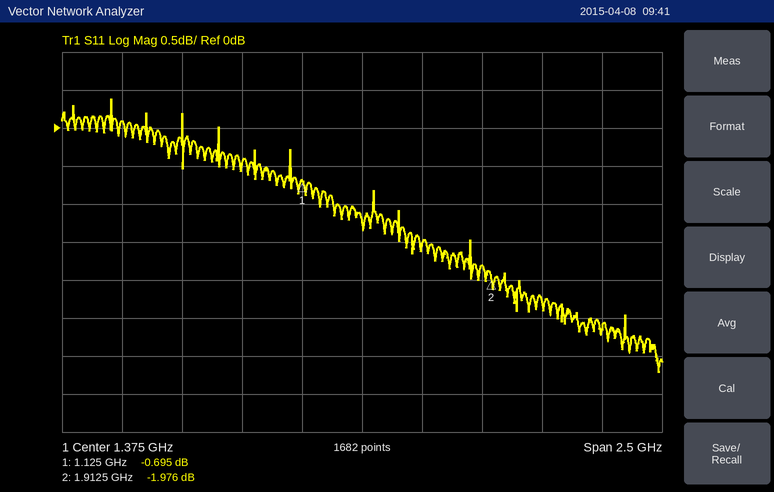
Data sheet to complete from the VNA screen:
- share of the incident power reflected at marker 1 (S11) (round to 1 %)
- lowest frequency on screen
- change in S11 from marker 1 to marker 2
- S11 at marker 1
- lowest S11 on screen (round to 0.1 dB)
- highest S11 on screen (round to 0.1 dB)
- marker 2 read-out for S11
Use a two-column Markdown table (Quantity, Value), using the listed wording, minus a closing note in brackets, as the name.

| Quantity | Value |
|---|---|
| share of the incident power reflected at marker 1 (S11) | 85 % |
| lowest frequency on screen | 125 MHz |
| change in S11 from marker 1 to marker 2 | -1.281 dB |
| S11 at marker 1 | -0.695 dB |
| lowest S11 on screen | -3.2 dB |
| highest S11 on screen | 0.4 dB |
| marker 2 read-out for S11 | -1.976 dB |
